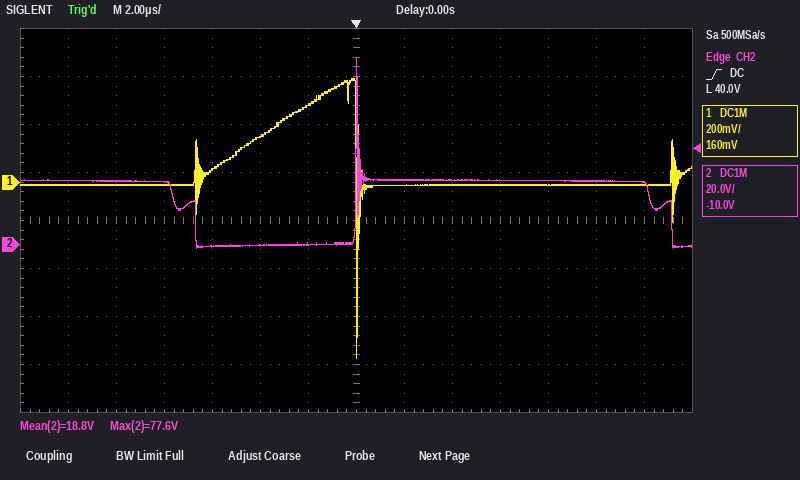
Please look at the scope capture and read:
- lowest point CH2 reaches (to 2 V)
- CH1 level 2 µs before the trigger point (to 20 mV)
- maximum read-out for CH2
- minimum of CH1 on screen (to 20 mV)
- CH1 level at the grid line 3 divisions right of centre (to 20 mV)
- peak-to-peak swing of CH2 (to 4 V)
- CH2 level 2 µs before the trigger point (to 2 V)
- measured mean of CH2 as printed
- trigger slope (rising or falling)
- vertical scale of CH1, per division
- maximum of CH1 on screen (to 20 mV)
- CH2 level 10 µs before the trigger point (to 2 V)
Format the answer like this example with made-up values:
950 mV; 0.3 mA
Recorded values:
-2 V; 320 mV; 77.6 V; -740 mV; -20 mV; 80 V; 0 V; 18.8 V; rising; 200 mV; 440 mV; 26 V
